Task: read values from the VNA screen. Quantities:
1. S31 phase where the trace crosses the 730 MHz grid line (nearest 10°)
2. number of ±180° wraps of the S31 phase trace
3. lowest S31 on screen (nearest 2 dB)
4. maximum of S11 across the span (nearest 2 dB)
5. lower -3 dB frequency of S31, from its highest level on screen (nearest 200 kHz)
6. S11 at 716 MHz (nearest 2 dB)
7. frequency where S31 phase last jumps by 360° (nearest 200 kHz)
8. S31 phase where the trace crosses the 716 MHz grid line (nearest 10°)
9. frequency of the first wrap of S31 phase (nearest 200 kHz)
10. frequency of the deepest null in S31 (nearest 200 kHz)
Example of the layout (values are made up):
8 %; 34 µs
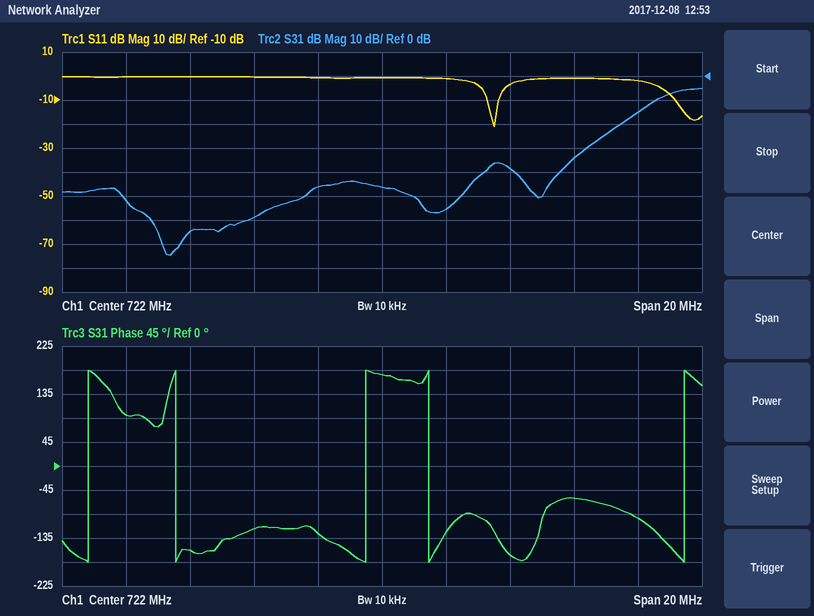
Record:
-100°; 5; -74 dB; 0 dB; 730.8 MHz; 0 dB; 731.4 MHz; -160°; 712.8 MHz; 715.4 MHz
